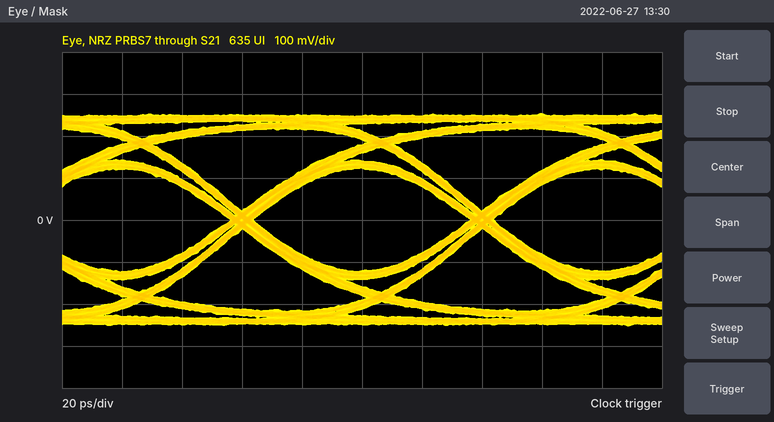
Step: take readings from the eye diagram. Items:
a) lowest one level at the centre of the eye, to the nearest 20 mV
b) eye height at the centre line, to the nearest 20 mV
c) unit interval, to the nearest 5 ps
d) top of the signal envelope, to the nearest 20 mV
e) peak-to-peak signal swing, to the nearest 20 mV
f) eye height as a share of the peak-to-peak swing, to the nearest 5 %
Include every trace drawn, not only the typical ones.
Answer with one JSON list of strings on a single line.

["120 mV", "240 mV", "80 ps", "260 mV", "500 mV", "50 %"]
